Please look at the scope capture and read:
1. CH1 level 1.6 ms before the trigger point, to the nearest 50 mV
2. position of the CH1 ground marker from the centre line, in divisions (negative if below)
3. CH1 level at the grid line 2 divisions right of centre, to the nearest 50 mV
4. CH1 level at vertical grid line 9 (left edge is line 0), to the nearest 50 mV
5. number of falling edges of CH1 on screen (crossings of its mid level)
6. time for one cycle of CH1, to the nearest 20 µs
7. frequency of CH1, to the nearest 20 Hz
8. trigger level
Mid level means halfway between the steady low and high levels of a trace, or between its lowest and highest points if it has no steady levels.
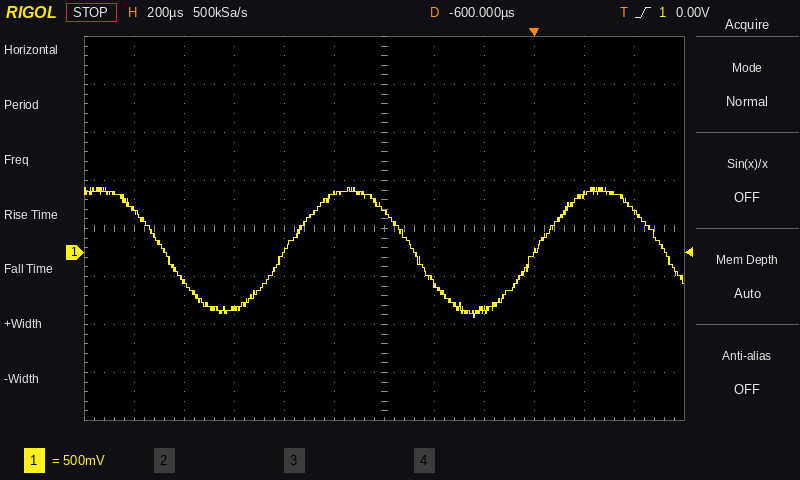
450 mV
-0.5 div
-600 mV
0 mV
3
1.00 ms
1.00 kHz
0.00 V
